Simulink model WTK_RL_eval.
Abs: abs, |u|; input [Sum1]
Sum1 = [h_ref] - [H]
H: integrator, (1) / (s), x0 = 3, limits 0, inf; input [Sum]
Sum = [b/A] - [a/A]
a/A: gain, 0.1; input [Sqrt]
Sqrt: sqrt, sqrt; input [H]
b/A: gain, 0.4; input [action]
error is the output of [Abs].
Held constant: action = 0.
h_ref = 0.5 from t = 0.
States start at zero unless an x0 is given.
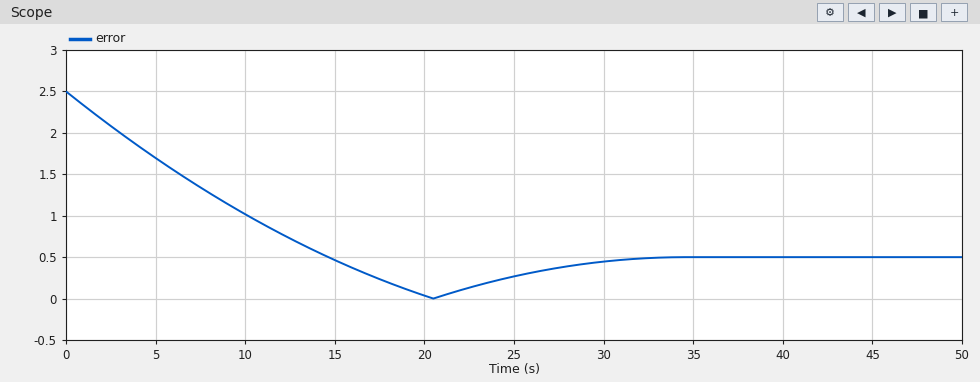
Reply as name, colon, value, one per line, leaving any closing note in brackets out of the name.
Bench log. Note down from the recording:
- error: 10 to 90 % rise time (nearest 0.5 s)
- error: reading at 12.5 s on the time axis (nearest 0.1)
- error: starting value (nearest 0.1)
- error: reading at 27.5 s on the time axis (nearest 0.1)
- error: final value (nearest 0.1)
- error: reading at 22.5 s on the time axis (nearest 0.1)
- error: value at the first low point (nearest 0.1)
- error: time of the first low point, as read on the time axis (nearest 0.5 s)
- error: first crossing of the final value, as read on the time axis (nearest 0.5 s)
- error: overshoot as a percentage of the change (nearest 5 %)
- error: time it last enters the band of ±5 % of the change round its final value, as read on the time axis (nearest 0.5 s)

error: 10 to 90 % rise time: 11.5 s
error: reading at 12.5 s on the time axis: 0.7
error: starting value: 2.5
error: reading at 27.5 s on the time axis: 0.4
error: final value: 0.5
error: reading at 22.5 s on the time axis: 0.1
error: value at the first low point: 0.0
error: time of the first low point, as read on the time axis: 20.5 s
error: first crossing of the final value, as read on the time axis: 14.5 s
error: overshoot as a percentage of the change: 25 %
error: time it last enters the band of ±5 % of the change round its final value, as read on the time axis: 28.5 s
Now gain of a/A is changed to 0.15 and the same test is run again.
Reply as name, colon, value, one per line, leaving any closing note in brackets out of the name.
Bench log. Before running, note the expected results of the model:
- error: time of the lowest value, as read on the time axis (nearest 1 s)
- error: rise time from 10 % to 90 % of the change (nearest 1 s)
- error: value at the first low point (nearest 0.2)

error: time of the lowest value, as read on the time axis: 14 s
error: rise time from 10 % to 90 % of the change: 8 s
error: value at the first low point: 0.0
